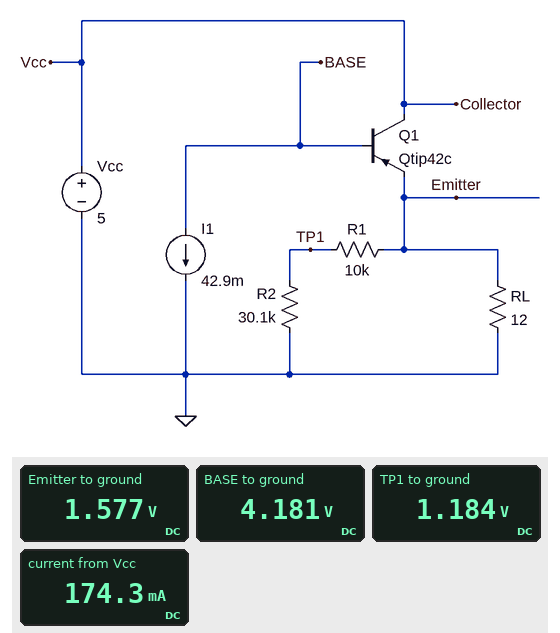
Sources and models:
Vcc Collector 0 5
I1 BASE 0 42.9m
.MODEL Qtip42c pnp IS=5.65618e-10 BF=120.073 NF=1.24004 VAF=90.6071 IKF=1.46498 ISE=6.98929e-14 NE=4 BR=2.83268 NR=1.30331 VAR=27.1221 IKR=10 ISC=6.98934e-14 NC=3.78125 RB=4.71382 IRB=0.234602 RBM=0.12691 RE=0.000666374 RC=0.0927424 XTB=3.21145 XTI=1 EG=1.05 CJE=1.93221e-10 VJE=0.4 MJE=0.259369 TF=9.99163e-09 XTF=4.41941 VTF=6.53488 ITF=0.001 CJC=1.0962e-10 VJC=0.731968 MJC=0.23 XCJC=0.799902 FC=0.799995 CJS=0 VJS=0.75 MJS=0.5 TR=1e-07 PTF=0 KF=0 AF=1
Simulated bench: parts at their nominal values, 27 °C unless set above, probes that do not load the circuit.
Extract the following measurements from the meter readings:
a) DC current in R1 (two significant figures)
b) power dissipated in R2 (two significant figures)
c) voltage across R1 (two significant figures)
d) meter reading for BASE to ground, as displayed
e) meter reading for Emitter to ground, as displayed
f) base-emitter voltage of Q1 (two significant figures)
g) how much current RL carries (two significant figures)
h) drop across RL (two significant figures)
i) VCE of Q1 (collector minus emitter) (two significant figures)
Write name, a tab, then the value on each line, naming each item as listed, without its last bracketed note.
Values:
DC current in R1	39 µA
power dissipated in R2	47 µW
voltage across R1	390 mV
meter reading for BASE to ground, as displayed	4.181 V
meter reading for Emitter to ground, as displayed	1.577 V
base-emitter voltage of Q1	2.6 V
how much current RL carries	130 mA
drop across RL	1.6 V
VCE of Q1 (collector minus emitter)	3.4 V
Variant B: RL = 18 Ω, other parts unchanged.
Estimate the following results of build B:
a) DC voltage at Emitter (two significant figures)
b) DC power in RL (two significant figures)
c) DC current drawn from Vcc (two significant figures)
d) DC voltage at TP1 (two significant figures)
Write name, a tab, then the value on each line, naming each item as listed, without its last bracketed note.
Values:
DC voltage at Emitter	2.3 V
DC power in RL	300 mW
DC current drawn from Vcc	170 mA
DC voltage at TP1	1.7 V
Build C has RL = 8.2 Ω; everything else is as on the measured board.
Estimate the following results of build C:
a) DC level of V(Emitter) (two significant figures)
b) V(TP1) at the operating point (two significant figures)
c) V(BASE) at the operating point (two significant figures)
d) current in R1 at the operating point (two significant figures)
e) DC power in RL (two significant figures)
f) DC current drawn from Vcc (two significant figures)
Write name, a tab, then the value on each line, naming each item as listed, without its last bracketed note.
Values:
DC level of V(Emitter)	1.1 V
V(TP1) at the operating point	820 mV
V(BASE) at the operating point	4.2 V
current in R1 at the operating point	27 µA
DC power in RL	150 mW
DC current drawn from Vcc	180 mA
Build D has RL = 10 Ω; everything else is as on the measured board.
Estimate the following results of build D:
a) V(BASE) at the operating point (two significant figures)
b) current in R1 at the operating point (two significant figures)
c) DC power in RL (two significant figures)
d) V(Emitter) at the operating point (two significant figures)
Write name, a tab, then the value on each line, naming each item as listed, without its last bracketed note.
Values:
V(BASE) at the operating point	4.2 V
current in R1 at the operating point	33 µA
DC power in RL	180 mW
V(Emitter) at the operating point	1.3 V
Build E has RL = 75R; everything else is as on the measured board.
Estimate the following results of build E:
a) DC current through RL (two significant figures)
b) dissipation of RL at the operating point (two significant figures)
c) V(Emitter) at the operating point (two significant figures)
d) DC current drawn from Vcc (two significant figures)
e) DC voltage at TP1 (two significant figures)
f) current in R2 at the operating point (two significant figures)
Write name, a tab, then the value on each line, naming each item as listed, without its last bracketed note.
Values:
DC current through RL	66 mA
dissipation of RL at the operating point	320 mW
V(Emitter) at the operating point	4.9 V
DC current drawn from Vcc	110 mA
DC voltage at TP1	3.7 V
current in R2 at the operating point	120 µA
